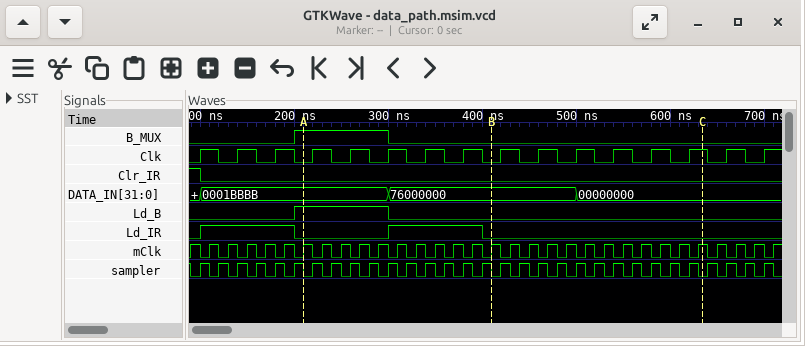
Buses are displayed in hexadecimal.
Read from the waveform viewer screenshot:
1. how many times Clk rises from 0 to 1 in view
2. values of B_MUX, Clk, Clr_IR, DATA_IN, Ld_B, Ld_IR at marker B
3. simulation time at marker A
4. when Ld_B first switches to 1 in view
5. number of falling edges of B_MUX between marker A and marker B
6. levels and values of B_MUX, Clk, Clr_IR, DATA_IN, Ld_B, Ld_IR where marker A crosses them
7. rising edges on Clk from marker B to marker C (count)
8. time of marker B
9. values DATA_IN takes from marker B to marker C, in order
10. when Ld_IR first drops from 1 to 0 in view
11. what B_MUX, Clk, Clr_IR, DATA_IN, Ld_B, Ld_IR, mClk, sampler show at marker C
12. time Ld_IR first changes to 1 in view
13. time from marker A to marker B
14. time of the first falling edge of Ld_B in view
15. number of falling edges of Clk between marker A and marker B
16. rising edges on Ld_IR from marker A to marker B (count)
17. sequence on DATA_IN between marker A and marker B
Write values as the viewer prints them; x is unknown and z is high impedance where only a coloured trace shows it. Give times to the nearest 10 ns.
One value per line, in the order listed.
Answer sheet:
16
B_MUX=0, Clk=0, Clr_IR=0, DATA_IN=76000000, Ld_B=0, Ld_IR=0
210 ns
200 ns
1
B_MUX=1, Clk=0, Clr_IR=0, DATA_IN=0001BBBB, Ld_B=1, Ld_IR=0
6
410 ns
76000000, 00000000
200 ns
B_MUX=0, Clk=1, Clr_IR=0, DATA_IN=00000000, Ld_B=0, Ld_IR=0, mClk=1, sampler=0
100 ns
200 ns
300 ns
5
1
0001BBBB, 76000000
